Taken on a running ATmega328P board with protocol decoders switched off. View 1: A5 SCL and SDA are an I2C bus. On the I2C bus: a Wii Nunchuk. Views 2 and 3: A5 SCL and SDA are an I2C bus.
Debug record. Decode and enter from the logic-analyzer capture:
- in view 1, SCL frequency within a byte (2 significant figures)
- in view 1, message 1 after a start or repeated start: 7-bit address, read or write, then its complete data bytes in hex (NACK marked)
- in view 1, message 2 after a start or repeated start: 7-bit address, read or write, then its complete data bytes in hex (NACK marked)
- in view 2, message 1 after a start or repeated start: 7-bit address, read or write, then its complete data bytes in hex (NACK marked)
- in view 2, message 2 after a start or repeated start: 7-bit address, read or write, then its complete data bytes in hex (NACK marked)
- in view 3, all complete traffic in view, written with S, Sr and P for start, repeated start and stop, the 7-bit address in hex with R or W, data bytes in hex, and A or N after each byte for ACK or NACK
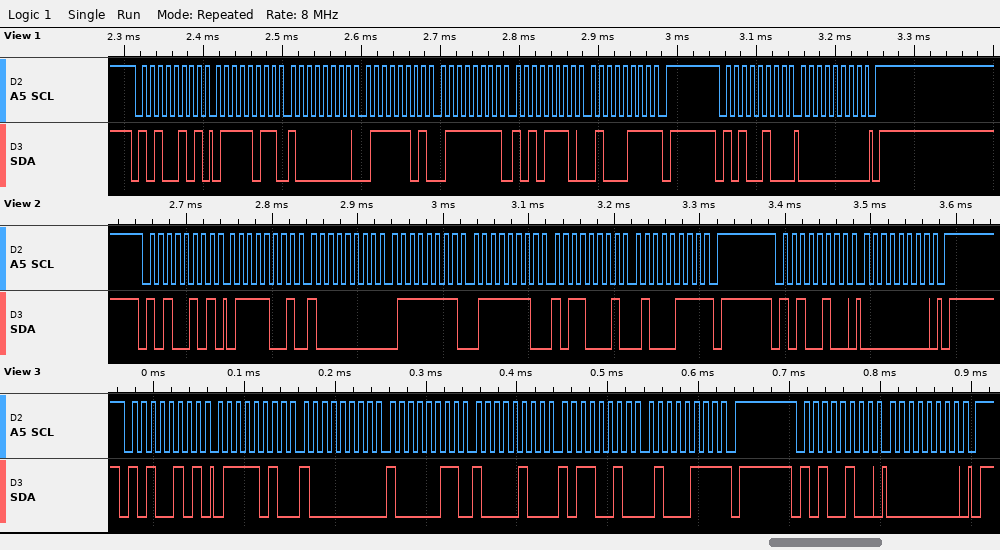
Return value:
100 kHz
0x52 read: 7B 80 7D 7F AE 47 NACK
0x52 write: 00
0x52 read: 79 80 7F 7E B1 47 NACK
0x52 write: 00
S 52R A 7A A 80 A 83 A 84 A B2 A 47 N P S 52W A 00 A P
